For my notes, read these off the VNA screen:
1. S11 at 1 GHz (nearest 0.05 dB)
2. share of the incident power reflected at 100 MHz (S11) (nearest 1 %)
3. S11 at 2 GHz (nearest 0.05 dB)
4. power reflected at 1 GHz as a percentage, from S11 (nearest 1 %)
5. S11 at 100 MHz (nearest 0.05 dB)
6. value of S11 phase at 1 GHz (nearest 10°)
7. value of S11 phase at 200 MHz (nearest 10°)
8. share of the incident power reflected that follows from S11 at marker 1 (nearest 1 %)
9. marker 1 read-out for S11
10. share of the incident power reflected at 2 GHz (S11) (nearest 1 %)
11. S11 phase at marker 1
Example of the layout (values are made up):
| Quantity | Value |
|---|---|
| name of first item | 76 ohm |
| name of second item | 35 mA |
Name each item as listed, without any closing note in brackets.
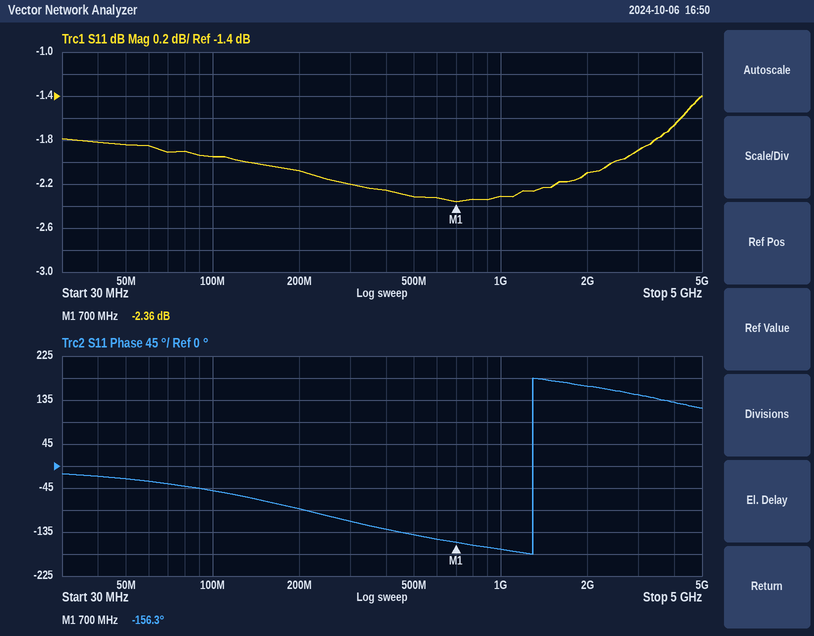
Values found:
| Quantity | Value |
|---|---|
| S11 at 1 GHz | -2.30 dB |
| share of the incident power reflected at 100 MHz (S11) | 64 % |
| S11 at 2 GHz | -2.10 dB |
| power reflected at 1 GHz as a percentage, from S11 | 59 % |
| S11 at 100 MHz | -1.95 dB |
| value of S11 phase at 1 GHz | -170° |
| value of S11 phase at 200 MHz | -90° |
| share of the incident power reflected that follows from S11 at marker 1 | 58 % |
| marker 1 read-out for S11 | -2.36 dB |
| share of the incident power reflected at 2 GHz (S11) | 62 % |
| S11 phase at marker 1 | -156.3° |
